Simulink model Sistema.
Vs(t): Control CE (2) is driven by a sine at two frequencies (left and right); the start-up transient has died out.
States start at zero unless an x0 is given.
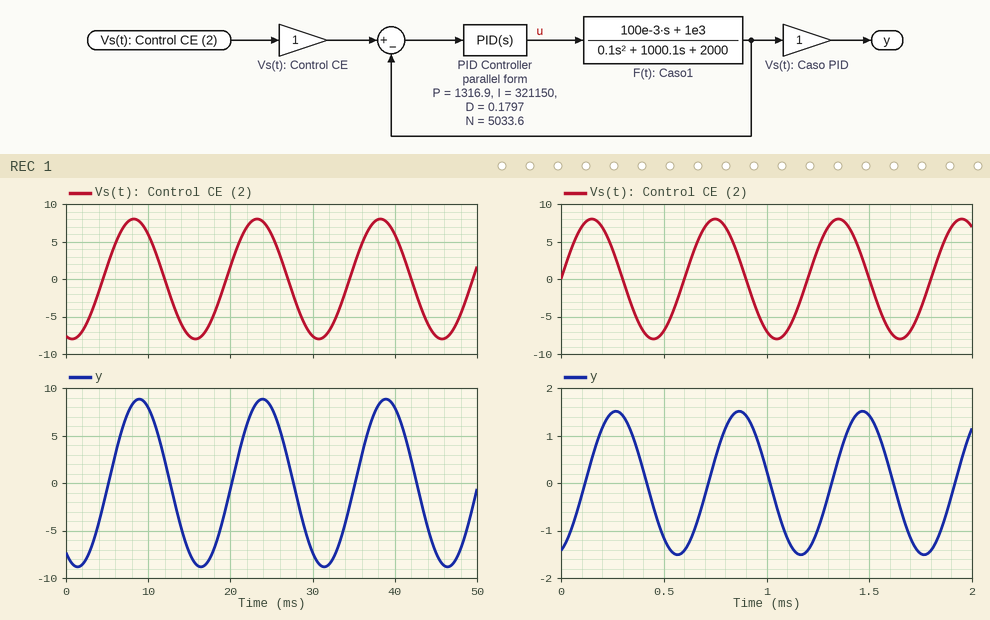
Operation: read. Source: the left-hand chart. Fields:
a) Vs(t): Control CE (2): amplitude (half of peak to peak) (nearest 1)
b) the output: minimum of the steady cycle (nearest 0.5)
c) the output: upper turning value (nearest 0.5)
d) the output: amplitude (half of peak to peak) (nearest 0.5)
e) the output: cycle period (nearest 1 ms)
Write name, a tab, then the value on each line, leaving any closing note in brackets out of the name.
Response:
Vs(t): Control CE (2): amplitude (half of peak to peak)	8
the output: minimum of the steady cycle	-9.0
the output: upper turning value	9.0
the output: amplitude (half of peak to peak)	9.0
the output: cycle period	15 ms
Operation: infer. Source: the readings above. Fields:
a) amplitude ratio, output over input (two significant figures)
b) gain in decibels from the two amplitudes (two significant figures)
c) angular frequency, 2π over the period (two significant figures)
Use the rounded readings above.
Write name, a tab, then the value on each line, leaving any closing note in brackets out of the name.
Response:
amplitude ratio, output over input	1.1
gain in decibels from the two amplitudes	1.0 dB
angular frequency, 2π over the period	0.42 rad/ms
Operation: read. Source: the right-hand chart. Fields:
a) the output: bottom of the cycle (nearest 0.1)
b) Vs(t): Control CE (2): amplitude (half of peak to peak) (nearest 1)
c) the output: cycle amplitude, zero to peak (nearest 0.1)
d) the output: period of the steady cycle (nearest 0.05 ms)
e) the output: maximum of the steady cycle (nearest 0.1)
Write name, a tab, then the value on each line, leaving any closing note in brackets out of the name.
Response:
the output: bottom of the cycle	-1.5
Vs(t): Control CE (2): amplitude (half of peak to peak)	8
the output: cycle amplitude, zero to peak	1.5
the output: period of the steady cycle	0.60 ms
the output: maximum of the steady cycle	1.5
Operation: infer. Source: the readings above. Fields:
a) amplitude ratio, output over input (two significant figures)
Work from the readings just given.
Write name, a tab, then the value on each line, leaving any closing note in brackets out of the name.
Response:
amplitude ratio, output over input	0.19
